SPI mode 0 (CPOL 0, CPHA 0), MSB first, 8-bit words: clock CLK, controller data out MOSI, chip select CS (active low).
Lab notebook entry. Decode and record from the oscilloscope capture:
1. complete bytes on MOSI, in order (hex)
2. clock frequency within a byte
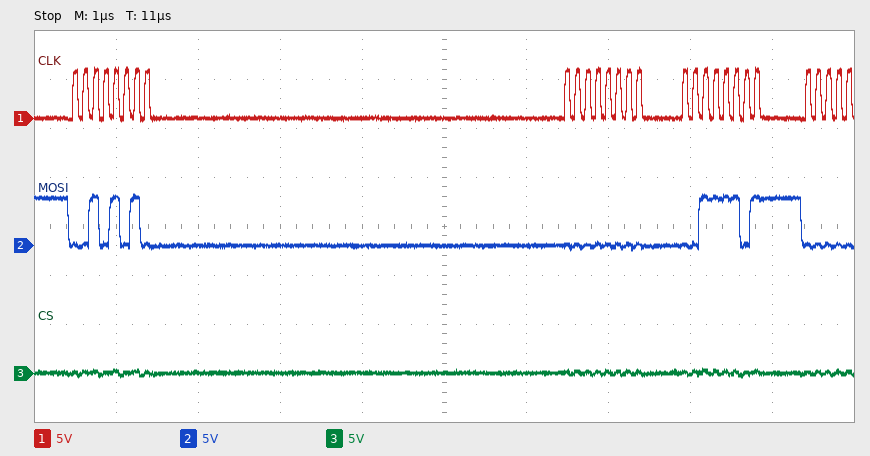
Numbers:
2A 00 3D
8 MHz
